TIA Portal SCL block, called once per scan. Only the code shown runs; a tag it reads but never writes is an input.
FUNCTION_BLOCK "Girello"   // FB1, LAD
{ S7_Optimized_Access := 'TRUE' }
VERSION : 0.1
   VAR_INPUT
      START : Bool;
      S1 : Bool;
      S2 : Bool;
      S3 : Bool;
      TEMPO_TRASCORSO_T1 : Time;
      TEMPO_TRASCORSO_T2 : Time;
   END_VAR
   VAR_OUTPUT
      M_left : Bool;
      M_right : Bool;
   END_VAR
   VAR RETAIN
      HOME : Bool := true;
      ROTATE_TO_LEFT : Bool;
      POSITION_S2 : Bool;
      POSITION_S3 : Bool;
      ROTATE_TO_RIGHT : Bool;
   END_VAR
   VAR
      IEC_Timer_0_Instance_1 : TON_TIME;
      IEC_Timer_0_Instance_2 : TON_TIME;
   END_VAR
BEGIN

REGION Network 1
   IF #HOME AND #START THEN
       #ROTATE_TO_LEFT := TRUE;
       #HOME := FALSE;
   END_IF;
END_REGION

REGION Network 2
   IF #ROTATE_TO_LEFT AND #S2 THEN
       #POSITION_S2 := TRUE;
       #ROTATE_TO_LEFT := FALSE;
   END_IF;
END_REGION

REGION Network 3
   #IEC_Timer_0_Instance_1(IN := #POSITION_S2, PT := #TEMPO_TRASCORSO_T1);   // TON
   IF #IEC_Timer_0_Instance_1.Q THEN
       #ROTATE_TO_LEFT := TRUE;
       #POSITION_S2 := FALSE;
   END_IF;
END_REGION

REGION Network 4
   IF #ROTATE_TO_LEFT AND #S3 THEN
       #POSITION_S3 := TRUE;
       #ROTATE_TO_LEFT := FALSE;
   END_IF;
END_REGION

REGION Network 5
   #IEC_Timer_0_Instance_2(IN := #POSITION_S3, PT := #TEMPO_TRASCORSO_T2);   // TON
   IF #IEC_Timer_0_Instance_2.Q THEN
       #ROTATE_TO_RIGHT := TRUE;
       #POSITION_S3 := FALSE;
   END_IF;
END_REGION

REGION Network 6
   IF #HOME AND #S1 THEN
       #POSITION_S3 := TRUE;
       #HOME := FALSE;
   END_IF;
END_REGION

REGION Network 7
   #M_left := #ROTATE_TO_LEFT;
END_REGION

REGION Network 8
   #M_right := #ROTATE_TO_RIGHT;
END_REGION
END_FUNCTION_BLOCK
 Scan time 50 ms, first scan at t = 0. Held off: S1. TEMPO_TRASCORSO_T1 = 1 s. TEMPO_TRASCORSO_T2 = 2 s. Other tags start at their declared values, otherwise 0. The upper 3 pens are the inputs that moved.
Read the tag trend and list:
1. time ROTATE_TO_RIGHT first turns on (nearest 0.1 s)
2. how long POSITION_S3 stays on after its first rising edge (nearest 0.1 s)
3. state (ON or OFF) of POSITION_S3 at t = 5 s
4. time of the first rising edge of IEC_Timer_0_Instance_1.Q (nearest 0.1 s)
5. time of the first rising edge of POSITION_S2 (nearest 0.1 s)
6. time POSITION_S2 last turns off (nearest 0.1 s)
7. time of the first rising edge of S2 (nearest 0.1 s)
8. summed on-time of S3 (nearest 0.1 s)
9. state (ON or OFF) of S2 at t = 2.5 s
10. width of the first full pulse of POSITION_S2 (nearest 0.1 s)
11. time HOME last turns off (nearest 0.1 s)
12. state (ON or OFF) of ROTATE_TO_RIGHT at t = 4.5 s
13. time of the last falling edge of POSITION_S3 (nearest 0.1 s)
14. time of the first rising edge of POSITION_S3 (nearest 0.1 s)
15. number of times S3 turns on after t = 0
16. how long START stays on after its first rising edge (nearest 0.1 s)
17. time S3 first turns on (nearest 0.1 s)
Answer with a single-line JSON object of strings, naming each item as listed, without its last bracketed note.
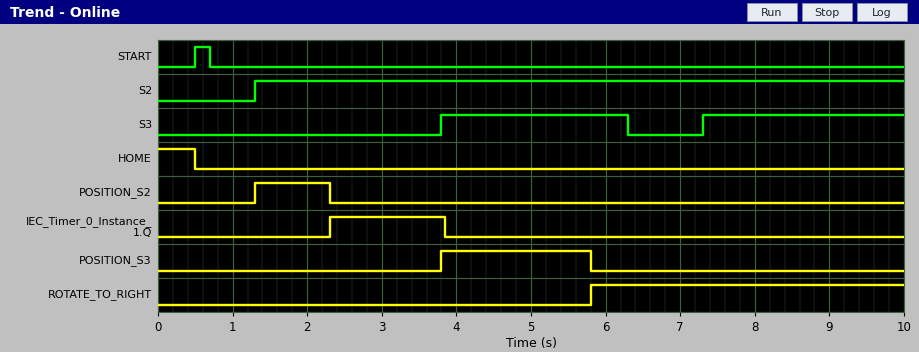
{"time ROTATE_TO_RIGHT first turns on": "5.8 s", "how long POSITION_S3 stays on after its first rising edge": "2.0 s", "state (ON or OFF) of POSITION_S3 at t = 5 s": "ON", "time of the first rising edge of IEC_Timer_0_Instance_1.Q": "2.3 s", "time of the first rising edge of POSITION_S2": "1.3 s", "time POSITION_S2 last turns off": "2.3 s", "time of the first rising edge of S2": "1.3 s", "summed on-time of S3": "5.2 s", "state (ON or OFF) of S2 at t = 2.5 s": "ON", "width of the first full pulse of POSITION_S2": "1.0 s", "time HOME last turns off": "0.5 s", "state (ON or OFF) of ROTATE_TO_RIGHT at t = 4.5 s": "OFF", "time of the last falling edge of POSITION_S3": "5.8 s", "time of the first rising edge of POSITION_S3": "3.8 s", "number of times S3 turns on after t = 0": "2", "how long START stays on after its first rising edge": "0.2 s", "time S3 first turns on": "3.8 s"}
